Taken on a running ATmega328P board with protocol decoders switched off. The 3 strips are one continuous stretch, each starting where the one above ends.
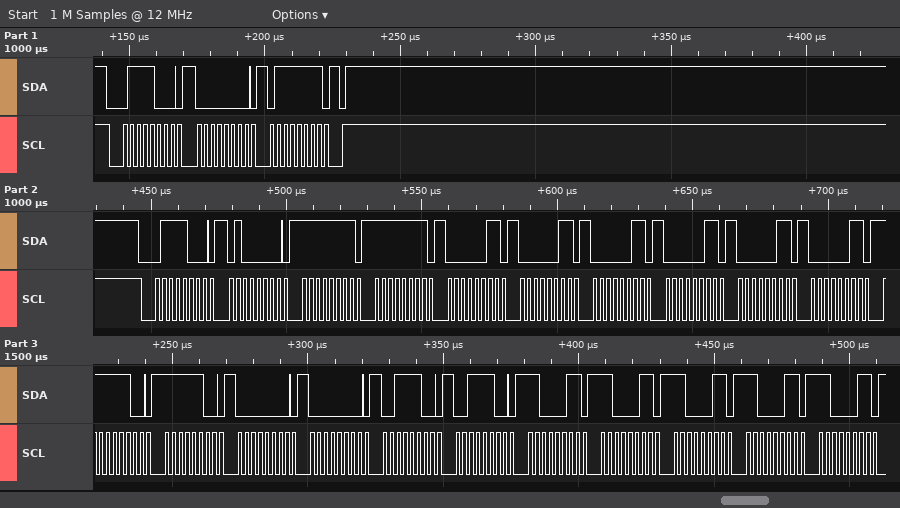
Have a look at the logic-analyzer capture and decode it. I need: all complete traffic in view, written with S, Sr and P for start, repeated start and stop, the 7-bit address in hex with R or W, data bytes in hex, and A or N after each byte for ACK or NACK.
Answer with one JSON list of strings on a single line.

["S 3CW A 00 A 7F A P S 3CW A 40 A FF A FF A 03 A 03 A 03 A 03 A 03 A 03 A FC A FC A 00 A 00 A 3C A 3C A C3 A C3 A C3 A C3 A C3 A"]
